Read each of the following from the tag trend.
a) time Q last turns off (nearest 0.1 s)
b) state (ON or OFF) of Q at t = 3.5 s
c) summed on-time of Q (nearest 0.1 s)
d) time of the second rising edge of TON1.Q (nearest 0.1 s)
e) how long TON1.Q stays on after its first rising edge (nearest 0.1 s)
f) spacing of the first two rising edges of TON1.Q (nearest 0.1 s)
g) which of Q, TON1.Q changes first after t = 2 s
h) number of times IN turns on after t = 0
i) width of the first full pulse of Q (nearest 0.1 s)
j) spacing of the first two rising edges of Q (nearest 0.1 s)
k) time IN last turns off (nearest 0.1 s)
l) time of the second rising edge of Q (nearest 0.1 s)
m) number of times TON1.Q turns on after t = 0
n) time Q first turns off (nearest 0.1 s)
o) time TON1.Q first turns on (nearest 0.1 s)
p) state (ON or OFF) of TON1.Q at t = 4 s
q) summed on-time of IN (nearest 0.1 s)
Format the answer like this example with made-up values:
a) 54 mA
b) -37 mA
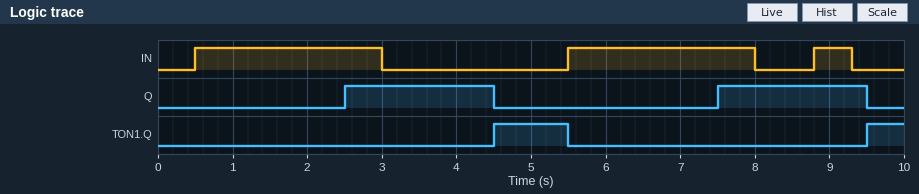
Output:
a) 9.5 s
b) ON
c) 4.0 s
d) 9.5 s
e) 1.0 s
f) 5.0 s
g) Q
h) 3
i) 2.0 s
j) 5.0 s
k) 9.3 s
l) 7.5 s
m) 2
n) 4.5 s
o) 4.5 s
p) OFF
q) 5.5 s
